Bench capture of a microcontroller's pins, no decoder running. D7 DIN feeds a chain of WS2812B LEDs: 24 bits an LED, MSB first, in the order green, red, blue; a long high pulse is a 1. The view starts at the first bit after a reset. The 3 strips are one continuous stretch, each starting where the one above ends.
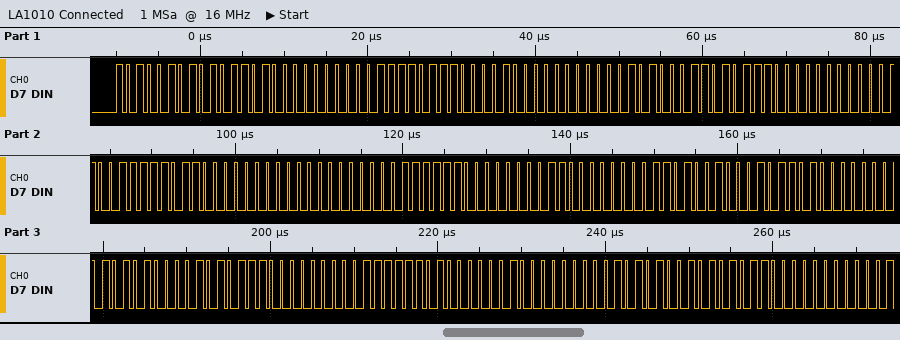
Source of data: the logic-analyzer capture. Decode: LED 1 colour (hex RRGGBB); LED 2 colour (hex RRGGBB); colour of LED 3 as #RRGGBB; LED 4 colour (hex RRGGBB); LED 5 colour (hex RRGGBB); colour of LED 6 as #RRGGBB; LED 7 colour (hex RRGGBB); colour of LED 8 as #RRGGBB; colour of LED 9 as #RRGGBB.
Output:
#5AA500
#847B00
#AE5100
#D82700
#FC0003
#D2002D
#A80057
#7E0081
#5400AB
